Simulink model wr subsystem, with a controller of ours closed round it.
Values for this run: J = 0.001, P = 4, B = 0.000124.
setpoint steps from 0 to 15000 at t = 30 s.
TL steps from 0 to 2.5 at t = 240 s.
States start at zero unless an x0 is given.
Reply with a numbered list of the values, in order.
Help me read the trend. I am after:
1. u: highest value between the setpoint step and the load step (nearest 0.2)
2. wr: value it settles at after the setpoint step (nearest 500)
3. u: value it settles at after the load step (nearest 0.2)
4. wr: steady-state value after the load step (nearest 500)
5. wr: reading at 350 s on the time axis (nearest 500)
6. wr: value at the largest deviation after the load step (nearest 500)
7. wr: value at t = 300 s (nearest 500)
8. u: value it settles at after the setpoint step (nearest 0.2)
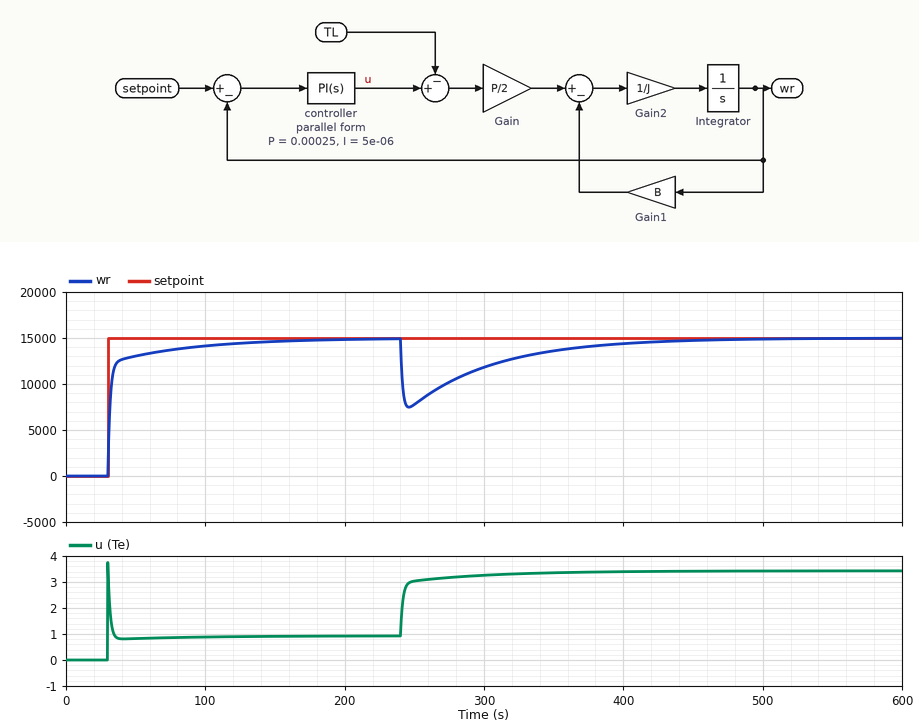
1. 3.8
2. 15000
3. 3.4
4. 15000
5. 13500
6. 7500
7. 12000
8. 1.0
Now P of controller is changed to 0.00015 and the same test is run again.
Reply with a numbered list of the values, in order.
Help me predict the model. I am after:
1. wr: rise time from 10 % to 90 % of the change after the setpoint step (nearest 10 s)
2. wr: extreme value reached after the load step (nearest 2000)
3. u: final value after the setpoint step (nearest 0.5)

1. 40 s
2. 4000
3. 1.0
